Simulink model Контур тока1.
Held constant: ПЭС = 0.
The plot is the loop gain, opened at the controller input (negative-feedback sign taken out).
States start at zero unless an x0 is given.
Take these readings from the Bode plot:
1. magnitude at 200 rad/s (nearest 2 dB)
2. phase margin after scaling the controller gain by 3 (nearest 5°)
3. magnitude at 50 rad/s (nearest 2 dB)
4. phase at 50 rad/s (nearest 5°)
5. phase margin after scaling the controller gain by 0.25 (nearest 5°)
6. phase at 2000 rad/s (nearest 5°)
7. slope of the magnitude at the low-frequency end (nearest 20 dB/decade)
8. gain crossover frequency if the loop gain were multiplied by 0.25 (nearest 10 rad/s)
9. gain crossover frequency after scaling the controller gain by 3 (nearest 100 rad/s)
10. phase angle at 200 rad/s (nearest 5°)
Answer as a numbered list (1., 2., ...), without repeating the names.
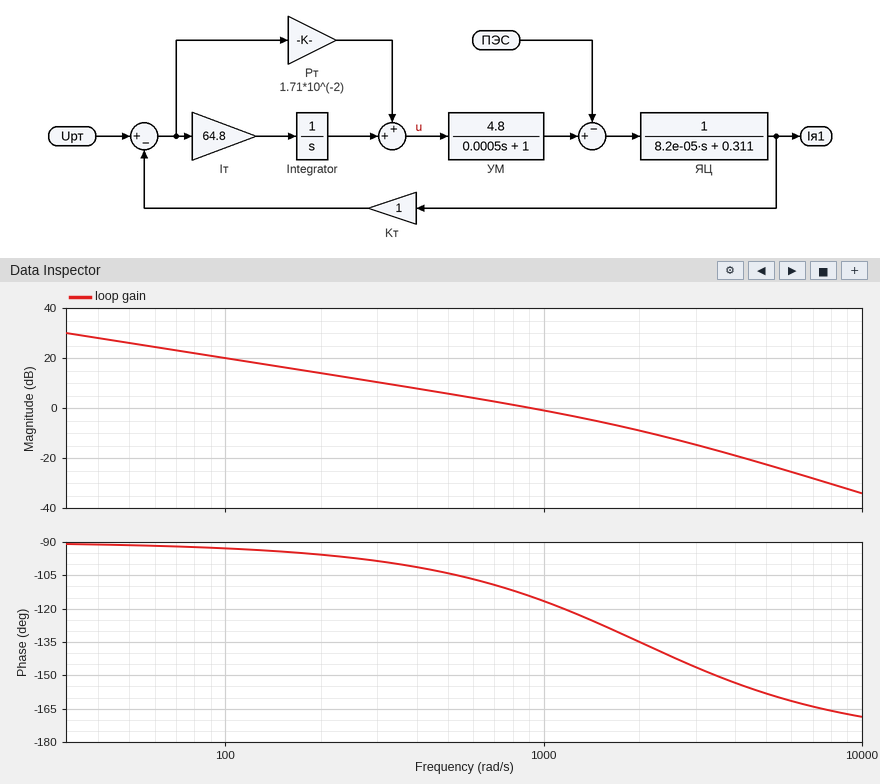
1. 14 dB
2. 45°
3. 26 dB
4. -90°
5. 85°
6. -135°
7. -20 dB/decade
8. 250 rad/s
9. 2100 rad/s
10. -95°
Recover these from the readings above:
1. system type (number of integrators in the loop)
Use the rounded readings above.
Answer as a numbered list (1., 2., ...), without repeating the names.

1. 1
